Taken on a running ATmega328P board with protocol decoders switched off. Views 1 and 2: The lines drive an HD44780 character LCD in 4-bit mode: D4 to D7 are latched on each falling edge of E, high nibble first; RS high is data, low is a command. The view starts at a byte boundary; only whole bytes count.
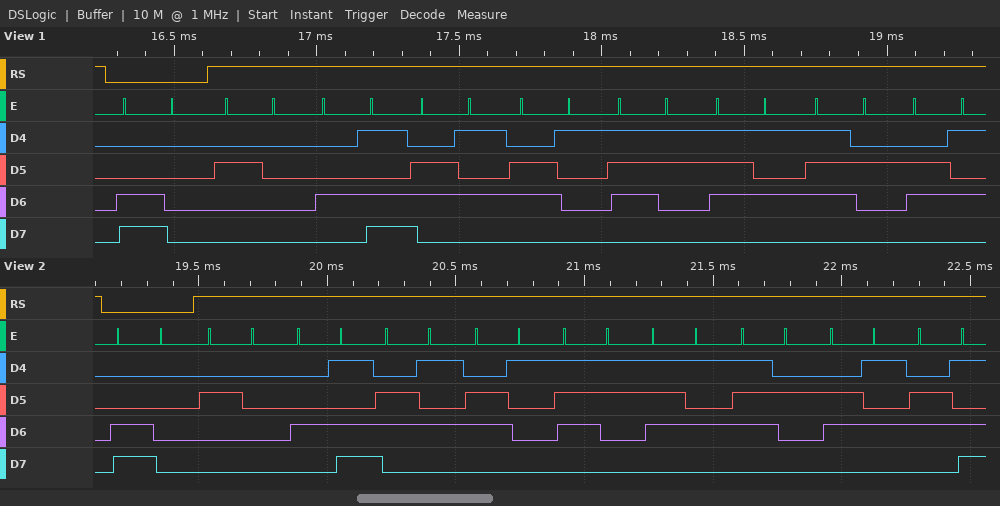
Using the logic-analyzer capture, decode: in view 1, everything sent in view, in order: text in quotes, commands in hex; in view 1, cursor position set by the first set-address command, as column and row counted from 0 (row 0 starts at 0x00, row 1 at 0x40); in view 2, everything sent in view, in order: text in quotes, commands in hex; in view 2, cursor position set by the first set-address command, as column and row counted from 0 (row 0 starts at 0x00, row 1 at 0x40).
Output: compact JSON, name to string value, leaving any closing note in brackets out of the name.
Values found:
{"in view 1, everything sent in view, in order: text in quotes, commands in hex": "0xC0 \" Measure\"", "in view 1, cursor position set by the first set-address command, as column and row counted from 0": "column 0, row 1", "in view 2, everything sent in view, in order: text in quotes, commands in hex": "0xC0 \" Measurem\"", "in view 2, cursor position set by the first set-address command, as column and row counted from 0": "column 0, row 1"}
